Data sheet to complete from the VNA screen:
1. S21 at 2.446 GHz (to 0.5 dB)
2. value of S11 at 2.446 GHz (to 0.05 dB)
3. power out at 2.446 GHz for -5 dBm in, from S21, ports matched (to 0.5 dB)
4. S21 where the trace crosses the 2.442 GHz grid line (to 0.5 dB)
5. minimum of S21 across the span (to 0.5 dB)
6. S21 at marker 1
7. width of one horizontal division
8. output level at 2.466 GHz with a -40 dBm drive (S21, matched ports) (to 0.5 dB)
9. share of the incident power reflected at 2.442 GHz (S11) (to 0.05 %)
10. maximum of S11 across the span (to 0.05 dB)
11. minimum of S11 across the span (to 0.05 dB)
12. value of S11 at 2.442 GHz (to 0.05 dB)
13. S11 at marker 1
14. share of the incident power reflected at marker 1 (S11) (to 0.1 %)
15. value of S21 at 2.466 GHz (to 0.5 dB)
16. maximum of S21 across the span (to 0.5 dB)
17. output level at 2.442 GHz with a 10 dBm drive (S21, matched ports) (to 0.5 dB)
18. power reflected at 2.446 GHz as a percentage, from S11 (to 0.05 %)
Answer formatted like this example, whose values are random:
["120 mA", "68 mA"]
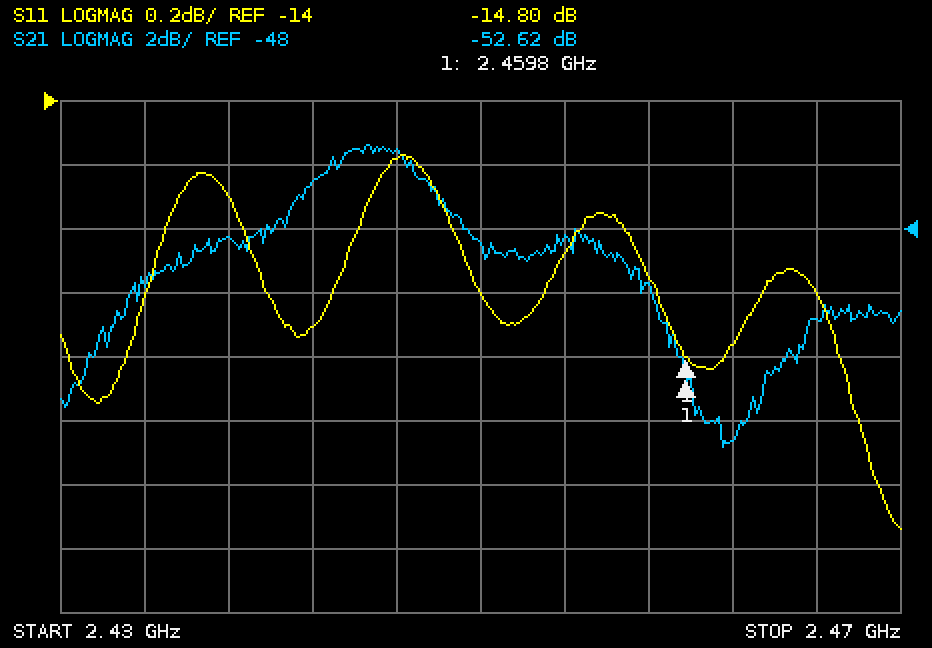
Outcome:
["-45.5 dB", "-14.20 dB", "-50.5 dBm", "-46.5 dB", "-55.0 dB", "-52.62 dB", "4 MHz", "-91.0 dBm", "3.40 %", "-14.15 dB", "-15.35 dB", "-14.70 dB", "-14.80 dB", "3.3 %", "-51.0 dB", "-45.5 dB", "-36.5 dBm", "3.80 %"]
